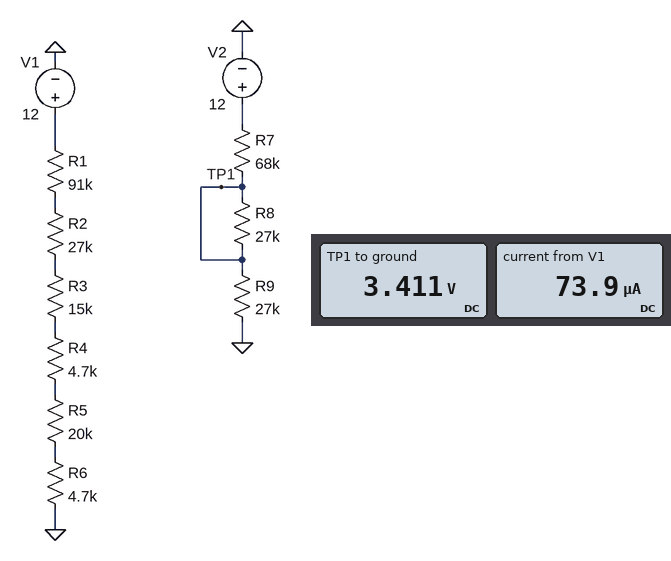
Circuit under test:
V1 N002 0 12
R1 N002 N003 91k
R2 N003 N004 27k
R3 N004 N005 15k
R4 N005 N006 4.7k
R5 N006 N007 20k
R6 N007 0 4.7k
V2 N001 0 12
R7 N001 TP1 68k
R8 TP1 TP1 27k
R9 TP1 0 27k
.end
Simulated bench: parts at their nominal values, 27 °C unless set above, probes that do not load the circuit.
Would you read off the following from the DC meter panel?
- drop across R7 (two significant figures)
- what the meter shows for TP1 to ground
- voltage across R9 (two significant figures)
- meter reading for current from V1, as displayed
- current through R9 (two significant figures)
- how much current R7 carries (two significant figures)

8.6 V
3.411 V
3.4 V
73.9 µA
130 µA
130 µA
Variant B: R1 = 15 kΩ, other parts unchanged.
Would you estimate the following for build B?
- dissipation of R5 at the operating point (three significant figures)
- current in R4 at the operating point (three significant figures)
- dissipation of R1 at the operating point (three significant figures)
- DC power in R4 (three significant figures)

386 µW
139 µA
289 µW
90.7 µW
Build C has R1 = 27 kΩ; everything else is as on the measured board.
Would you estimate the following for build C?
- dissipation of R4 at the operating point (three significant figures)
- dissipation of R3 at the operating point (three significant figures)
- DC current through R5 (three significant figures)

69.9 µW
223 µW
122 µA
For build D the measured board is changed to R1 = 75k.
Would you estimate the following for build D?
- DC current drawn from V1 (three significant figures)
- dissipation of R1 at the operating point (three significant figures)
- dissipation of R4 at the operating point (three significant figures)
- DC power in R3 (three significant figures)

82.0 µA
504 µW
31.6 µW
101 µW
